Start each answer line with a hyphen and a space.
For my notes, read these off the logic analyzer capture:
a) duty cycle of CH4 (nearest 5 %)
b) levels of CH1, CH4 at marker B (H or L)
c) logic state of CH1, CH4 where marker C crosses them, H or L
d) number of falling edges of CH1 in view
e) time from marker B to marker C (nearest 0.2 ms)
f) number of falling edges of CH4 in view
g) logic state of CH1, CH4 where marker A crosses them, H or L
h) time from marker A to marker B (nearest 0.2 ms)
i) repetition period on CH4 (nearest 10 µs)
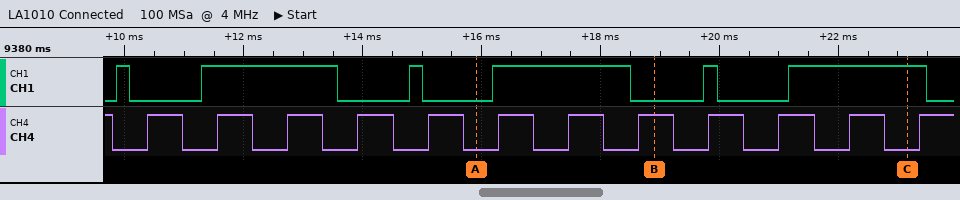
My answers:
- 50 %
- CH1=L, CH4=H
- CH1=H, CH4=L
- 6
- 4.2 ms
- 12
- CH1=L, CH4=L
- 3 ms
- 1180 µs
